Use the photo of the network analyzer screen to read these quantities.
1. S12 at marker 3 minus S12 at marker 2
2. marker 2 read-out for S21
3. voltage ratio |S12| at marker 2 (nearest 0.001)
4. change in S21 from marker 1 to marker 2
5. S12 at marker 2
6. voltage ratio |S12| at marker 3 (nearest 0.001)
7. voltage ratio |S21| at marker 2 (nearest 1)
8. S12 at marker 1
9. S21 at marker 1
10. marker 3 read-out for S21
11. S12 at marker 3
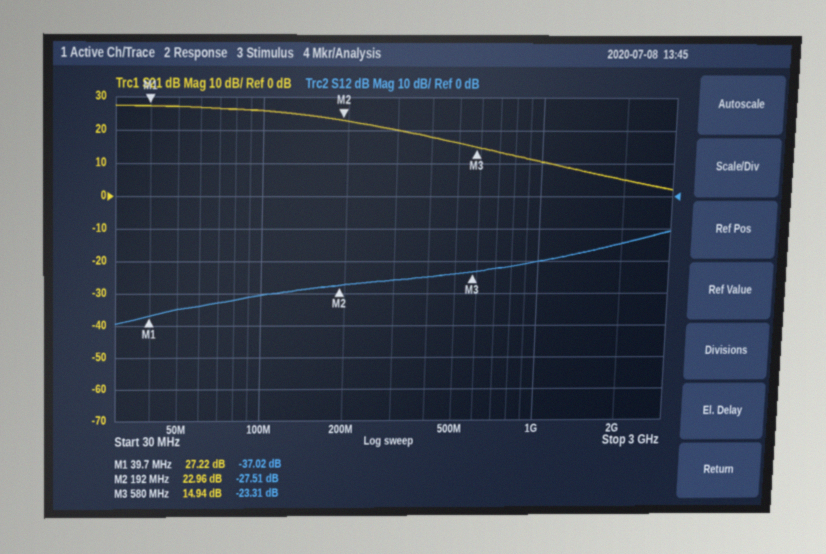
4.20 dB
22.96 dB
0.042
-4.26 dB
-27.51 dB
0.068
14
-37.02 dB
27.22 dB
14.94 dB
-23.31 dB
